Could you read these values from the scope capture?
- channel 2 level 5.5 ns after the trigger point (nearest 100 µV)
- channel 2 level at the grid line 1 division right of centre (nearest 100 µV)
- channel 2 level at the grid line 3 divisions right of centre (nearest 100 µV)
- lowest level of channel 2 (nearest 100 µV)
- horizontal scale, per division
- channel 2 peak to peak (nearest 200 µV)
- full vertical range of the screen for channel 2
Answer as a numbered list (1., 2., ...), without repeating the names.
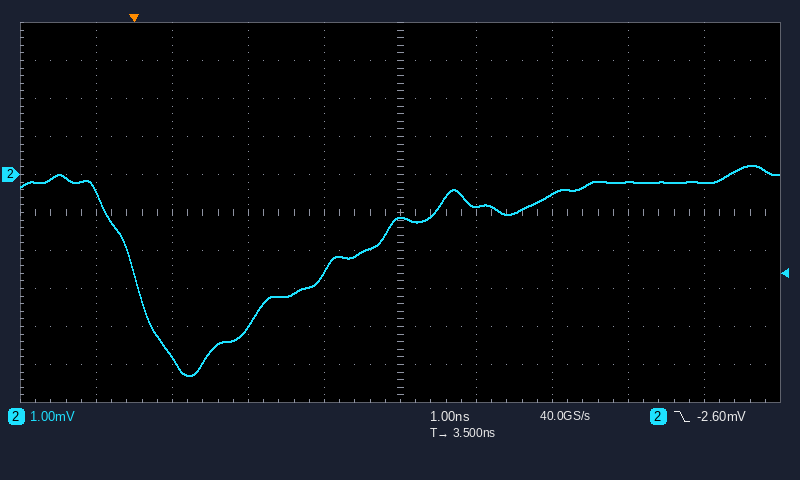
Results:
1. -500 µV
2. -800 µV
3. -200 µV
4. -5.3 mV
5. 1 ns
6. 5.6 mV
7. 10 mV
